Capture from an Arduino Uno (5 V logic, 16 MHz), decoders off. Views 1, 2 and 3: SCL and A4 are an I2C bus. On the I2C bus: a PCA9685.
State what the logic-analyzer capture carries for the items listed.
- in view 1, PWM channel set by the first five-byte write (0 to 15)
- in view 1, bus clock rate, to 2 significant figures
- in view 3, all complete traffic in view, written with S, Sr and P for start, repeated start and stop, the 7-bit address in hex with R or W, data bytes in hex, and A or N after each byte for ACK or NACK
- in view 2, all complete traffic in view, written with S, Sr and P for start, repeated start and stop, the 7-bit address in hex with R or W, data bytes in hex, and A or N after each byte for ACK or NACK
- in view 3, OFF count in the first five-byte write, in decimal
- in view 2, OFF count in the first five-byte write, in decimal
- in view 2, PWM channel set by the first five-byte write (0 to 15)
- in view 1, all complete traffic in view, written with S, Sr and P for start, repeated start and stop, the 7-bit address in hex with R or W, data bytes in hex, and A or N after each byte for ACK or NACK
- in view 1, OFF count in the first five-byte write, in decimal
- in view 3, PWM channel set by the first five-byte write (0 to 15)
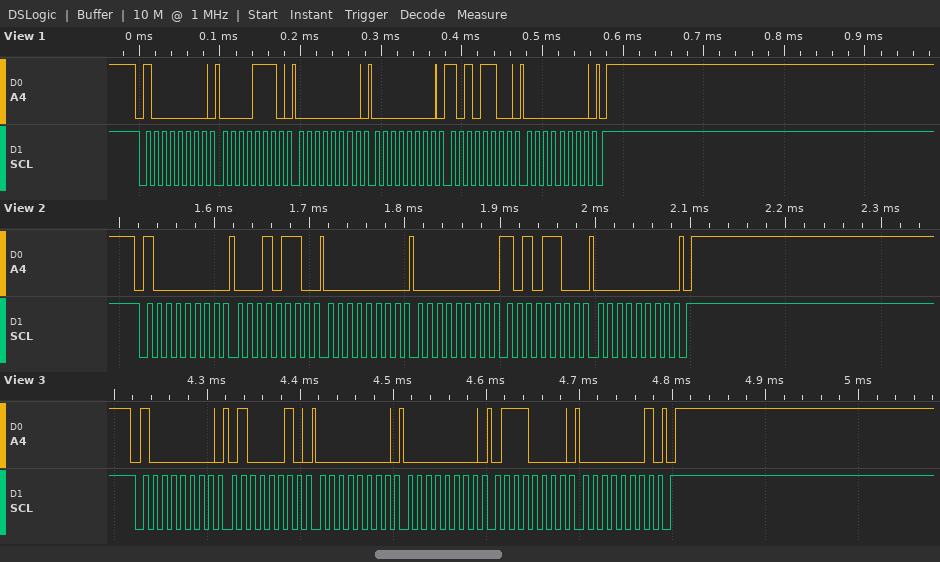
2
100 kHz
S 40W A 42 A 00 A 00 A 70 A 01 A P
S 40W A 16 A 00 A 00 A AC A 00 A P
368
172
4
S 40W A 0E A 00 A 00 A AC A 00 A P
172
15
